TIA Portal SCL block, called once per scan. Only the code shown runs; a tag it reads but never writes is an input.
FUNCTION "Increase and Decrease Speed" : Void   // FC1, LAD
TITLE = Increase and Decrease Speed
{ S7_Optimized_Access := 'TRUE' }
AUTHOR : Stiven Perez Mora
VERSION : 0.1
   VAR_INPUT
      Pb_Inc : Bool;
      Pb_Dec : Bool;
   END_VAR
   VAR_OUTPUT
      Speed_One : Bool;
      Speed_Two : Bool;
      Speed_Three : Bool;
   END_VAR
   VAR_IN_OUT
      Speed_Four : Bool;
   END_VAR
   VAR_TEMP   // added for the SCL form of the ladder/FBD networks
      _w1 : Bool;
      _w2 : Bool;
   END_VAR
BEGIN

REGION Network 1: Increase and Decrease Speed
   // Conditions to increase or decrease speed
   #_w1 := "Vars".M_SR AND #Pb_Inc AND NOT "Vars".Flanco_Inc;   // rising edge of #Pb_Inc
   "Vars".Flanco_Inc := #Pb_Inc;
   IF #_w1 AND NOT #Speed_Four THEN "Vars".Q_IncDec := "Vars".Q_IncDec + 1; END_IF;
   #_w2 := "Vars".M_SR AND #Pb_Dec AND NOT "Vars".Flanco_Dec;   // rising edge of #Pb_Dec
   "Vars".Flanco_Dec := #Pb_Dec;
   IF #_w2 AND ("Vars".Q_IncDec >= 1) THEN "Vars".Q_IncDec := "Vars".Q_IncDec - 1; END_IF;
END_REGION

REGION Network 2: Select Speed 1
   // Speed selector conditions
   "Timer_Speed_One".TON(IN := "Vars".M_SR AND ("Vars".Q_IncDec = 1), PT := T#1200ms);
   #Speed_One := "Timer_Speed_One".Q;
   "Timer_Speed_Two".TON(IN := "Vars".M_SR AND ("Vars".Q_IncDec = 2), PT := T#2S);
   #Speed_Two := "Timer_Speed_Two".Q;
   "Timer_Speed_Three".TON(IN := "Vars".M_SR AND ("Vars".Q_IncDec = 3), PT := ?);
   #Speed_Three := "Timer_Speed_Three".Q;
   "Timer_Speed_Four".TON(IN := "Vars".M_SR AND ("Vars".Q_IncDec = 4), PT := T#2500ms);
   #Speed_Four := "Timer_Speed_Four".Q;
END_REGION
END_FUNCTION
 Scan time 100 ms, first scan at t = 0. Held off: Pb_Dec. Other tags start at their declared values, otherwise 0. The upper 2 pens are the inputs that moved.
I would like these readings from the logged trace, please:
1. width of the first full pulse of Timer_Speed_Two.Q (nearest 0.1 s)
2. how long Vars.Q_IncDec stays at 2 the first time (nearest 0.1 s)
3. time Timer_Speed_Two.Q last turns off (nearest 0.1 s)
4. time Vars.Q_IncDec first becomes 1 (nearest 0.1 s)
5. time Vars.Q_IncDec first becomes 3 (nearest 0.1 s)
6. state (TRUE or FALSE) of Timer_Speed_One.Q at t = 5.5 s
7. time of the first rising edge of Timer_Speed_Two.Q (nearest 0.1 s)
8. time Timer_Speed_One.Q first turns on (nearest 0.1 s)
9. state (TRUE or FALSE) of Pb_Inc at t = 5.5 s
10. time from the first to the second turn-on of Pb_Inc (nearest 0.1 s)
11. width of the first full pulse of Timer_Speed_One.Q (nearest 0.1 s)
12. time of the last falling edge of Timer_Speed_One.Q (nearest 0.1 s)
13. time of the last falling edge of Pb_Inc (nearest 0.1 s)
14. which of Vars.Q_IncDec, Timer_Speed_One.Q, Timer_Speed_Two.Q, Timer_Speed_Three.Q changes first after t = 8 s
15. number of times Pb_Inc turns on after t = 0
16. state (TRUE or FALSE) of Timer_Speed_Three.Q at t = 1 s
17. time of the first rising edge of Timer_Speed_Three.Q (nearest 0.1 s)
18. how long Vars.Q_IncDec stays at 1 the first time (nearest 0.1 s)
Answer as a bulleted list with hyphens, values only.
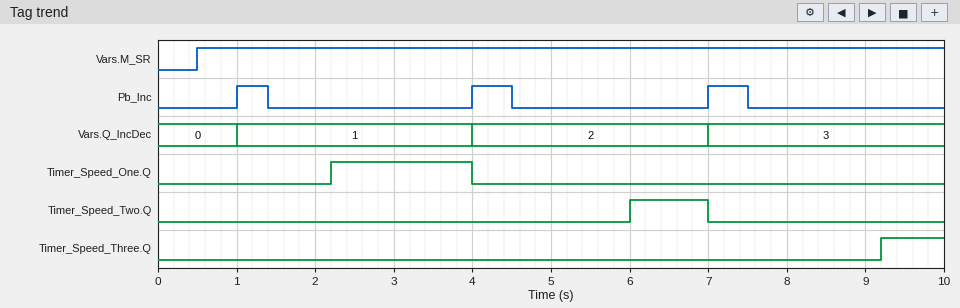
- 1.0 s
- 3.0 s
- 7.0 s
- 1.0 s
- 7.0 s
- FALSE
- 6.0 s
- 2.2 s
- FALSE
- 3.0 s
- 1.8 s
- 4.0 s
- 7.5 s
- Timer_Speed_Three.Q
- 3
- FALSE
- 9.2 s
- 3.0 s
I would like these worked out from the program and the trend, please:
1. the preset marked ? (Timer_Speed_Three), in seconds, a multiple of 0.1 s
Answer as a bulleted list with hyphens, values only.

- 2.2 s
